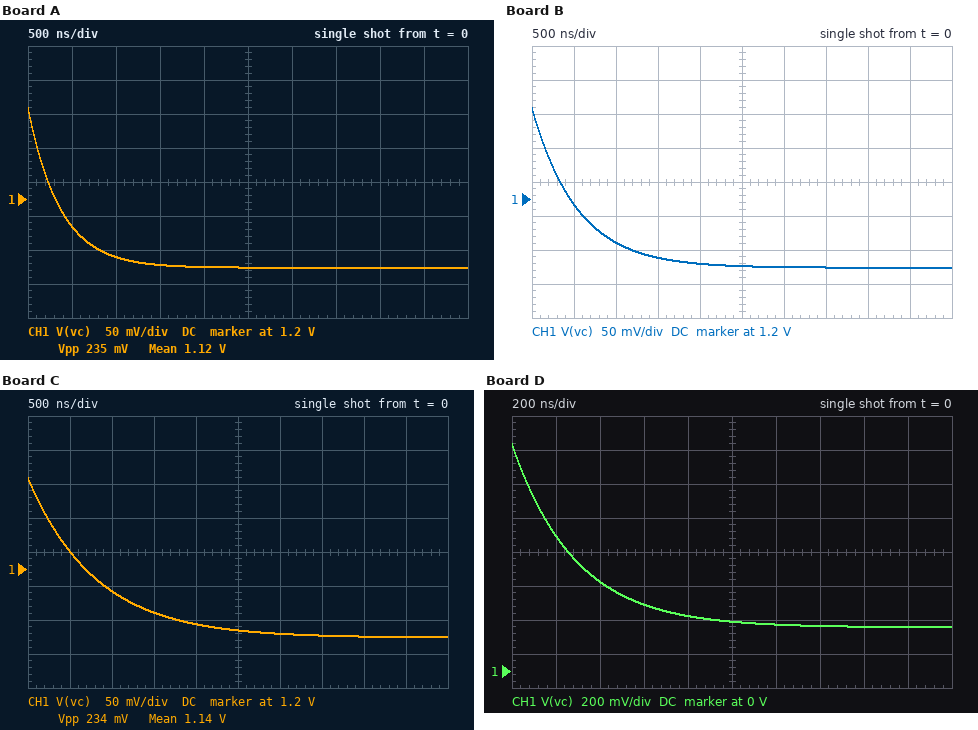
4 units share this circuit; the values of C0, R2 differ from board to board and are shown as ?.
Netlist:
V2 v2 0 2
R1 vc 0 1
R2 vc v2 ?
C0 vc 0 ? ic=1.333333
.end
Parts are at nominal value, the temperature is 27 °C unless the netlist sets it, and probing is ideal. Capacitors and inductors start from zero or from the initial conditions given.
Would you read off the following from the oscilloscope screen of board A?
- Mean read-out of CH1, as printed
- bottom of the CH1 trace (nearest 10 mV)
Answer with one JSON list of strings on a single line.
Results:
["1.12 V", "1.10 V"]
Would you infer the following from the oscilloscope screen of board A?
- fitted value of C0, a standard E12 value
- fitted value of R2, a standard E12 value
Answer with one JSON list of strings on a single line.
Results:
["820 nF", "0.82 Ω"]
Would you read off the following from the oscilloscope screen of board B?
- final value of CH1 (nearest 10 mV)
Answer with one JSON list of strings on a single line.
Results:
["1.10 V"]
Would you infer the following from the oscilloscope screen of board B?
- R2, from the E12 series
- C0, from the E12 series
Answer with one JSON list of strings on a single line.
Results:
["0.82 Ω", "1.2 µF"]
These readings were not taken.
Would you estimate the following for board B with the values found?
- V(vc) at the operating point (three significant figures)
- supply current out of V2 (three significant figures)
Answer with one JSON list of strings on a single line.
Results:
["1.10 V", "1.10 A"]
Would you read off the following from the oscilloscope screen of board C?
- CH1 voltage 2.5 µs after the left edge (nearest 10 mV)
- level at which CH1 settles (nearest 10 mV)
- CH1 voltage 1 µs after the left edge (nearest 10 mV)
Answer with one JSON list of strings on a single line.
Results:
["1.11 V", "1.10 V", "1.17 V"]
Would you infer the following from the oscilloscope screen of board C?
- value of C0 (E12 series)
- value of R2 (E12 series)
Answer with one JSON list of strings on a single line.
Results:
["1.8 µF", "0.82 Ω"]
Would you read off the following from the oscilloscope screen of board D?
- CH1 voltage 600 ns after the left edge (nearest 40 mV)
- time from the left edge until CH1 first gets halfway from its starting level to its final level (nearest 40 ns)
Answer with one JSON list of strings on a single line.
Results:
["400 mV", "200 ns"]
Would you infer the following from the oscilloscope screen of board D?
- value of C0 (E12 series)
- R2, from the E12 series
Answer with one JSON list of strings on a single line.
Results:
["330 nF", "6.8 Ω"]
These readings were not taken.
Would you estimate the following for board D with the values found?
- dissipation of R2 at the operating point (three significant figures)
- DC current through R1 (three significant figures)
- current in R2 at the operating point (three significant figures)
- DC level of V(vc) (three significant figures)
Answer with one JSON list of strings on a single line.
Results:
["447 mW", "256 mA", "256 mA", "256 mV"]
